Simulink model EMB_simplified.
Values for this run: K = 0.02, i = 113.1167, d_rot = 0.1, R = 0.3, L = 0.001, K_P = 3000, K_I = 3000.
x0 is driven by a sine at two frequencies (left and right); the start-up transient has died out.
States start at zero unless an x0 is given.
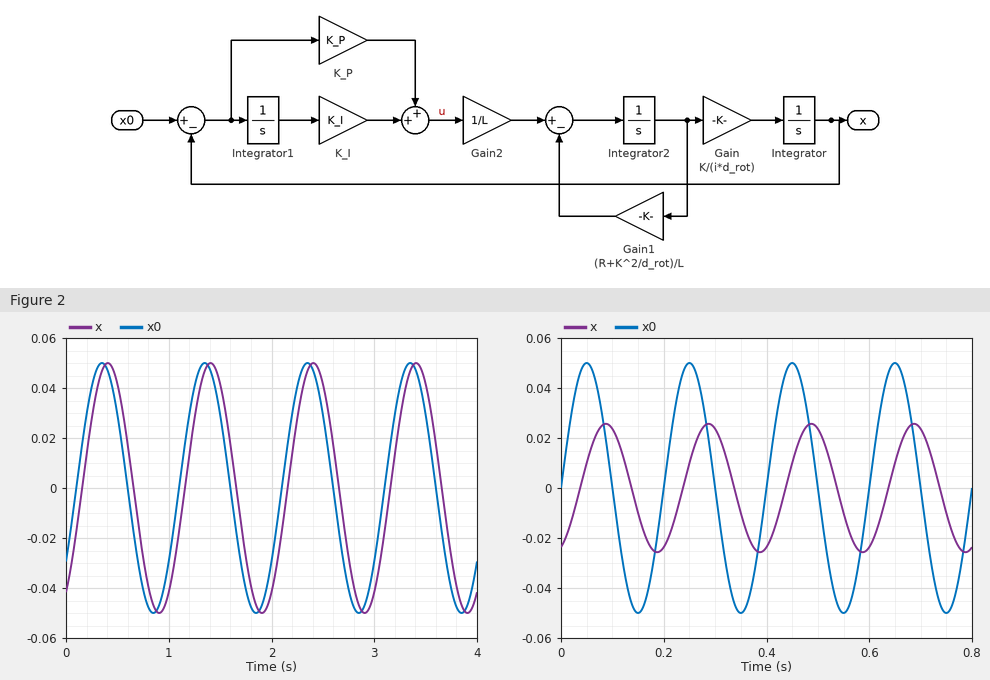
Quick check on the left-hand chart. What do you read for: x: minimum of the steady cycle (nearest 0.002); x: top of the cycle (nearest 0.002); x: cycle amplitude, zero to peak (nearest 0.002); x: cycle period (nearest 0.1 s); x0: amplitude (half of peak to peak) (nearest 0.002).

-0.050
0.050
0.050
1.0 s
0.050
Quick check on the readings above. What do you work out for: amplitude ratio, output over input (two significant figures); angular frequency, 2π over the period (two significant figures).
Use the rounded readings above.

1.0
6.3 rad/s
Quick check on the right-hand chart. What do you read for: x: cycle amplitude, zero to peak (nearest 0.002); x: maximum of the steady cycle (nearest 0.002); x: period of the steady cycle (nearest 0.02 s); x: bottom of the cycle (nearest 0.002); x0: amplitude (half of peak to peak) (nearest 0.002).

0.026
0.026
0.20 s
-0.026
0.050
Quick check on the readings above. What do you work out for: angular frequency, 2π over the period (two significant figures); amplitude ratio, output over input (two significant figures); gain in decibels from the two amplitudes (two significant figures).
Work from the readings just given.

31 rad/s
0.52
-5.7 dB
